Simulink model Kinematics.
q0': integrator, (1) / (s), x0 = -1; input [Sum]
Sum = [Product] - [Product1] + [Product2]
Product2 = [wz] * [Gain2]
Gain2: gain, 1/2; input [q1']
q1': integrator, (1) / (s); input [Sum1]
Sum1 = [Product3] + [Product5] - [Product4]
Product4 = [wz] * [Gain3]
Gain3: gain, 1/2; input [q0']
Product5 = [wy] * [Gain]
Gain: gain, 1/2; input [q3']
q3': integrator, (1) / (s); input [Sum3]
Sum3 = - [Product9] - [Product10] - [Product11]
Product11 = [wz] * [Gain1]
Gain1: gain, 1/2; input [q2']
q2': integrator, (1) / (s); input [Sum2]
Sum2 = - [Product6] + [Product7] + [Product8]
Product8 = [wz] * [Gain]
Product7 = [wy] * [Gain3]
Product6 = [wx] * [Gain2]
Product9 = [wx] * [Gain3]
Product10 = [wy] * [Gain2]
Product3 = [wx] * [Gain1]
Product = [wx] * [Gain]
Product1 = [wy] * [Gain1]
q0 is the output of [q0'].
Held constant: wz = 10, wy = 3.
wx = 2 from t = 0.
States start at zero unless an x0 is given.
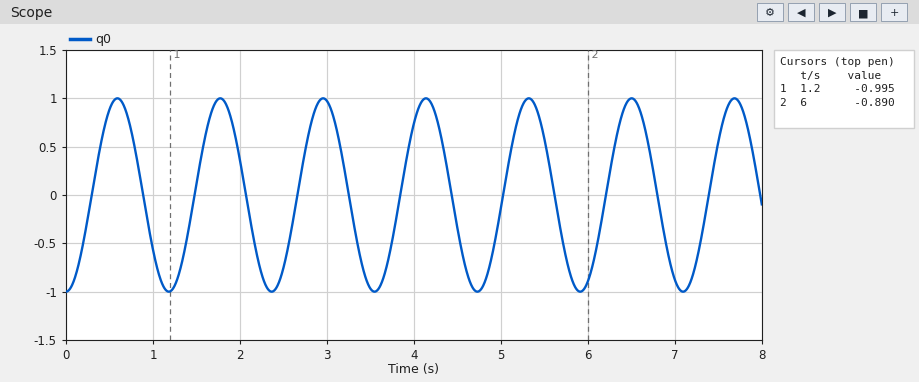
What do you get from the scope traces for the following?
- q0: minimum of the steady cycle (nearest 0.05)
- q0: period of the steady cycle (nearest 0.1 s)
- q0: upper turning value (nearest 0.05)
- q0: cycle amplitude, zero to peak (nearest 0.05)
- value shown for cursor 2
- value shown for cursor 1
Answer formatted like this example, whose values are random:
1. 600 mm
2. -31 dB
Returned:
1. -1.00
2. 1.2 s
3. 1.00
4. 1.00
5. -0.890
6. -0.995
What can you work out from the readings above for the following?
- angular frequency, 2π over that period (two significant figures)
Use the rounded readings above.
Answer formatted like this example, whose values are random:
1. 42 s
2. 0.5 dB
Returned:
1. 5.2 rad/s
